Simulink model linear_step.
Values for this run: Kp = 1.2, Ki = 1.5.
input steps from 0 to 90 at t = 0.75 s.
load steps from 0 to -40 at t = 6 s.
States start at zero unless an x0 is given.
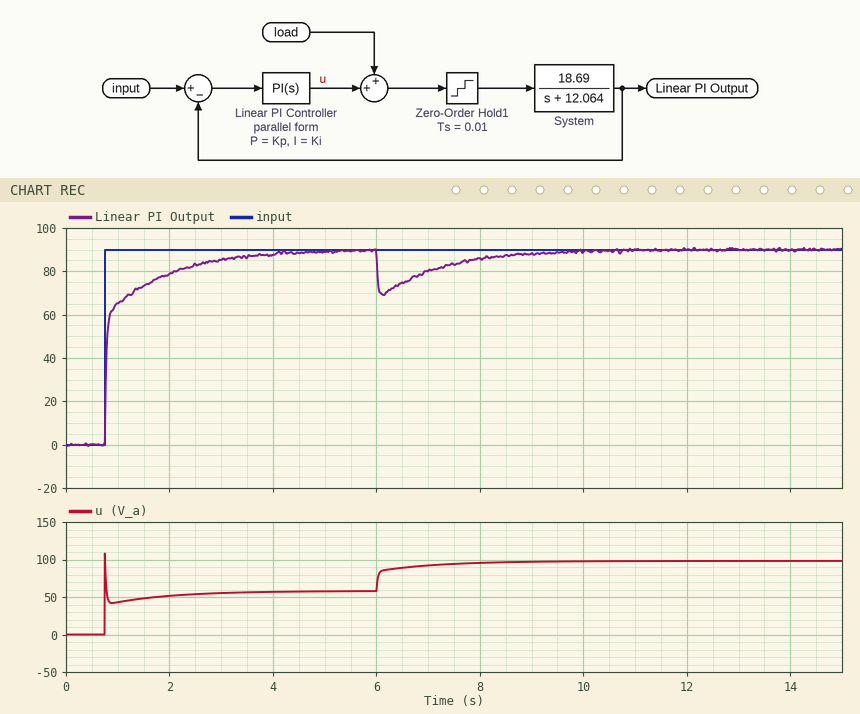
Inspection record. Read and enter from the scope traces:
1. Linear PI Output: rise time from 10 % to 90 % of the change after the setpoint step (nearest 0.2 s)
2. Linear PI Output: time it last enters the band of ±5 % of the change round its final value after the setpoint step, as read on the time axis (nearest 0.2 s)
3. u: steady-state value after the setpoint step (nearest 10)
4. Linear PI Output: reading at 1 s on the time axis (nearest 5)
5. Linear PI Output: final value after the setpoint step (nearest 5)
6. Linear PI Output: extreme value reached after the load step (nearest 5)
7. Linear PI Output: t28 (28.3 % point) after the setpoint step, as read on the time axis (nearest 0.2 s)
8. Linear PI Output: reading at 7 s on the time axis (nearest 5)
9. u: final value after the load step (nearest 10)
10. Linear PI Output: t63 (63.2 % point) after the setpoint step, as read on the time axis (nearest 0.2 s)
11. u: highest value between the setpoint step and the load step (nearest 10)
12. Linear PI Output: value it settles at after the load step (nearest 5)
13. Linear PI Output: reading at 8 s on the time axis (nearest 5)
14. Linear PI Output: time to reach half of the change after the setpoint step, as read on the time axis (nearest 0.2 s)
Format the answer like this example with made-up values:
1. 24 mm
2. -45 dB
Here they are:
1. 1.4 s
2. 3.0 s
3. 60
4. 65
5. 90
6. 70
7. 0.8 s
8. 80
9. 100
10. 0.8 s
11. 110
12. 90
13. 85
14. 0.8 s
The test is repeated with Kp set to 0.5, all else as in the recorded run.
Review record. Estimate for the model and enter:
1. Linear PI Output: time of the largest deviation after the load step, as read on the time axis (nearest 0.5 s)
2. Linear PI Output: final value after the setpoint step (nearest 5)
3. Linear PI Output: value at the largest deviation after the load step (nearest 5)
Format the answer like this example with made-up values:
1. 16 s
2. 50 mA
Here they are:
1. 6.0 s
2. 90
3. 60
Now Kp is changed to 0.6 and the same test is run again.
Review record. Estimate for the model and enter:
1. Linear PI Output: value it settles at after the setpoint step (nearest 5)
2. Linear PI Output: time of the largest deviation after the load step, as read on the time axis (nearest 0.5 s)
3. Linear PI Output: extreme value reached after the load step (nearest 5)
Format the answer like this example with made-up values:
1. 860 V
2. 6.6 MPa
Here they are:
1. 90
2. 6.0 s
3. 60
